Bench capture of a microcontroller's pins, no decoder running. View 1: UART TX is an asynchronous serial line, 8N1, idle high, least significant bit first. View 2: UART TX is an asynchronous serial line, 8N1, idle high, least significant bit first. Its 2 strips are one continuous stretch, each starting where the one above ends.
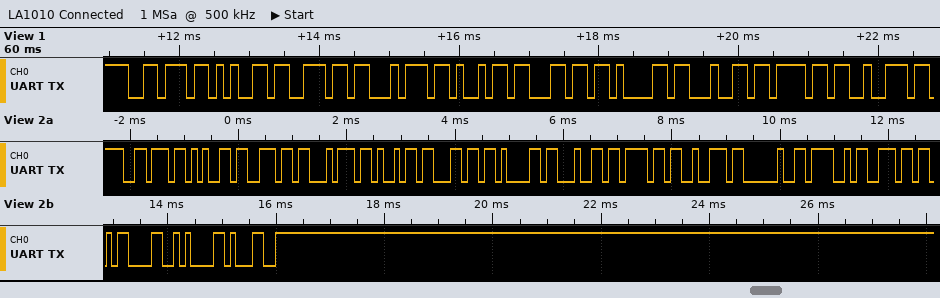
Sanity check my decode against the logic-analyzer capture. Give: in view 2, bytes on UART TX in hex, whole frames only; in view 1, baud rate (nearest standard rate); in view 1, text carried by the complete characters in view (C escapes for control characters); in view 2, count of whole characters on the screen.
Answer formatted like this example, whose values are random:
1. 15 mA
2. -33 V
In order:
1. 0x76 0x65 0x6E 0x74 0x69 0x6C 0x61 0x64 0x6F 0x72 0x20 0x4F 0x6E 0x0D 0x0A 0x31
2. 9600 baud
3. "ventilador"
4. 16
